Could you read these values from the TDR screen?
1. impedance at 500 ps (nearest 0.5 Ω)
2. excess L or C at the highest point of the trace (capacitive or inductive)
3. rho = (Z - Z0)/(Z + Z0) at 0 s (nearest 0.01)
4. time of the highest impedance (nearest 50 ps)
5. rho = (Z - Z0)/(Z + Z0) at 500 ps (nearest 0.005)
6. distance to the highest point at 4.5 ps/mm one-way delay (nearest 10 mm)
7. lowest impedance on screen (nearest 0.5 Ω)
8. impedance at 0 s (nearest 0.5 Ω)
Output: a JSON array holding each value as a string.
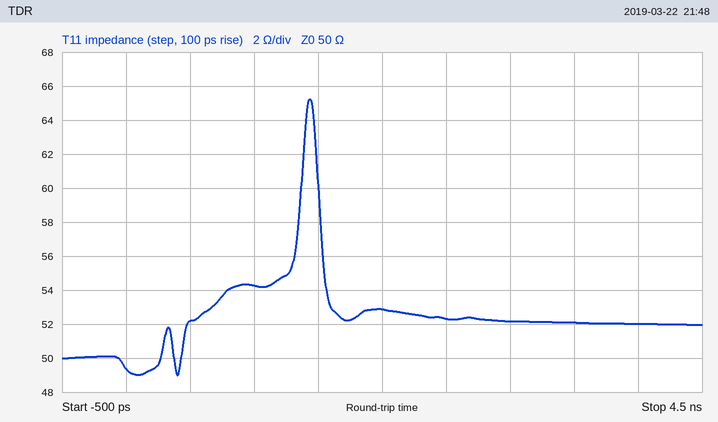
["52.0 Ω", "inductive", "-0.01", "1.45 ns", "+0.020", "160 mm", "49.0 Ω", "49.5 Ω"]
